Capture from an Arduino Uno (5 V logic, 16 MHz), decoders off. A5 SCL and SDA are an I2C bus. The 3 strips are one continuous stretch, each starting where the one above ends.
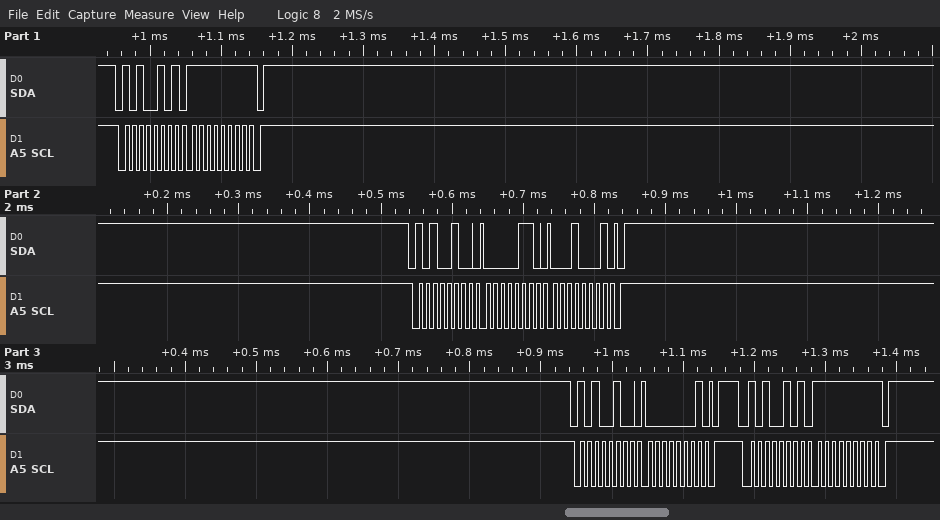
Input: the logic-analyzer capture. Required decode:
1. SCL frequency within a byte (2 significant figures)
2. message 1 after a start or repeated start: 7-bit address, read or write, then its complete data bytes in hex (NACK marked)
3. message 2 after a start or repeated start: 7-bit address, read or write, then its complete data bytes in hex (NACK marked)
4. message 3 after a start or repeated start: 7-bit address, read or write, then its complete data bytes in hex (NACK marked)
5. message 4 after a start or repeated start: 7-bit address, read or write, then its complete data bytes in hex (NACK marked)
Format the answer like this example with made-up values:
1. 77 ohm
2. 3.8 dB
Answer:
1. 100 kHz
2. 0x52 read: FF NACK
3. 0x52 write: 06 11
4. 0x52 write: 01
5. 0x52 read: FF NACK
